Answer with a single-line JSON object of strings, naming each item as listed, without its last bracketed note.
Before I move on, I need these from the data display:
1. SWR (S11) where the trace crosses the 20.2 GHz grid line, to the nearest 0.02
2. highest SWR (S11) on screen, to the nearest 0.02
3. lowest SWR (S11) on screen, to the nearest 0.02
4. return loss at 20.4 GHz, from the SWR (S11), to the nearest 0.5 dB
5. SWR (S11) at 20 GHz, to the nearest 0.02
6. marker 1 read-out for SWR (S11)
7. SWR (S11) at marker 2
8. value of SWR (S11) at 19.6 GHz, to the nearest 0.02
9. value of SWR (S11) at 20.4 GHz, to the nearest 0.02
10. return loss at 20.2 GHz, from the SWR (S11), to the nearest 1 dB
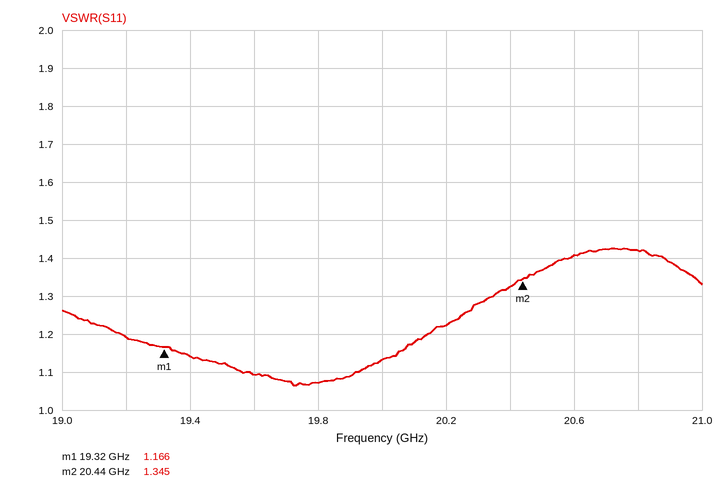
{"SWR (S11) where the trace crosses the 20.2 GHz grid line, to the nearest 0.02": "1.22", "highest SWR (S11) on screen, to the nearest 0.02": "1.42", "lowest SWR (S11) on screen, to the nearest 0.02": "1.06", "return loss at 20.4 GHz, from the SWR (S11), to the nearest 0.5 dB": "17.0 dB", "SWR (S11) at 20 GHz, to the nearest 0.02": "1.14", "marker 1 read-out for SWR": "1.166", "SWR (S11) at marker 2": "1.345", "value of SWR (S11) at 19.6 GHz, to the nearest 0.02": "1.10", "value of SWR (S11) at 20.4 GHz, to the nearest 0.02": "1.32", "return loss at 20.2 GHz, from the SWR (S11), to the nearest 1 dB": "20 dB"}
